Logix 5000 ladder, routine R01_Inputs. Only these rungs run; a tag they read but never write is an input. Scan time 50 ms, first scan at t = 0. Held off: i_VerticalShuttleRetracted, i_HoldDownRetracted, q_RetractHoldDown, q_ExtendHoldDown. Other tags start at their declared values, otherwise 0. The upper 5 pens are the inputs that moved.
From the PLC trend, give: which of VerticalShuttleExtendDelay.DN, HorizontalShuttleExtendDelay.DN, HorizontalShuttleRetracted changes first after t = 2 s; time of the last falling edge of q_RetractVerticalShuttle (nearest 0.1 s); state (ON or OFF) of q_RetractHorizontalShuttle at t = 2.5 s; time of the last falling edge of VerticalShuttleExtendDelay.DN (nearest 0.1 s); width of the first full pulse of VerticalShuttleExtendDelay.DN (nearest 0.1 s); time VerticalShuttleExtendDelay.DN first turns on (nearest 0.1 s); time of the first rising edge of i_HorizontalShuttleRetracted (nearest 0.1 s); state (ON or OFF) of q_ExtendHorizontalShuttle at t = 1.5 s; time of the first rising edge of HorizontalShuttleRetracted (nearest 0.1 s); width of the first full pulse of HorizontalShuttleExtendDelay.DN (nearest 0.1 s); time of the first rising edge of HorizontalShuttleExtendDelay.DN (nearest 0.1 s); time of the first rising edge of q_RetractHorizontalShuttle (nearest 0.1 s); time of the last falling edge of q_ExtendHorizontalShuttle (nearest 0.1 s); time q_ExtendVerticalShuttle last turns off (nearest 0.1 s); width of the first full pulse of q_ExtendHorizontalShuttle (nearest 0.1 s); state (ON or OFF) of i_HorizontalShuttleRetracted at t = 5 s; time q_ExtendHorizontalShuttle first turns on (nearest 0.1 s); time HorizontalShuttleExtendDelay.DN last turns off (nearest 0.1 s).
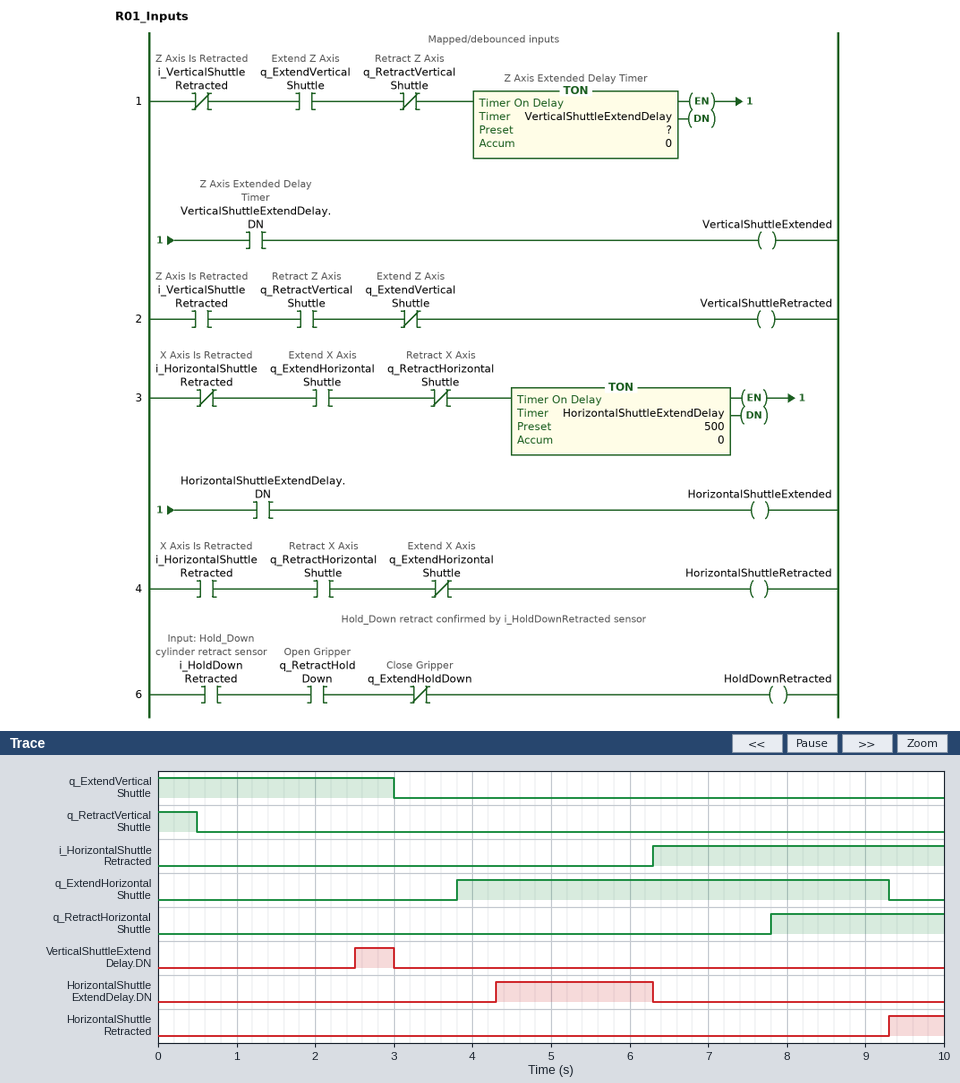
VerticalShuttleExtendDelay.DN
0.5 s
OFF
3.0 s
0.5 s
2.5 s
6.3 s
OFF
9.3 s
2.0 s
4.3 s
7.8 s
9.3 s
3.0 s
5.5 s
OFF
3.8 s
6.3 s
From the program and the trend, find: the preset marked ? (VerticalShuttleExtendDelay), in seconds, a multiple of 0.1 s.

2.0 s
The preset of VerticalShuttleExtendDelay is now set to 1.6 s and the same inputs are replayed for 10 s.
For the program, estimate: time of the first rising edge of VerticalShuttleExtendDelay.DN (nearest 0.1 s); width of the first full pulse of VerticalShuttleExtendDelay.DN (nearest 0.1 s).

2.1 s
0.9 s
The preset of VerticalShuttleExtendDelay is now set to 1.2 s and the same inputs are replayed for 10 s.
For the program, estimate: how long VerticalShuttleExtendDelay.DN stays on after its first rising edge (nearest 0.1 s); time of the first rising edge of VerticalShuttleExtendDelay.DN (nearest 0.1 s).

1.3 s
1.7 s
